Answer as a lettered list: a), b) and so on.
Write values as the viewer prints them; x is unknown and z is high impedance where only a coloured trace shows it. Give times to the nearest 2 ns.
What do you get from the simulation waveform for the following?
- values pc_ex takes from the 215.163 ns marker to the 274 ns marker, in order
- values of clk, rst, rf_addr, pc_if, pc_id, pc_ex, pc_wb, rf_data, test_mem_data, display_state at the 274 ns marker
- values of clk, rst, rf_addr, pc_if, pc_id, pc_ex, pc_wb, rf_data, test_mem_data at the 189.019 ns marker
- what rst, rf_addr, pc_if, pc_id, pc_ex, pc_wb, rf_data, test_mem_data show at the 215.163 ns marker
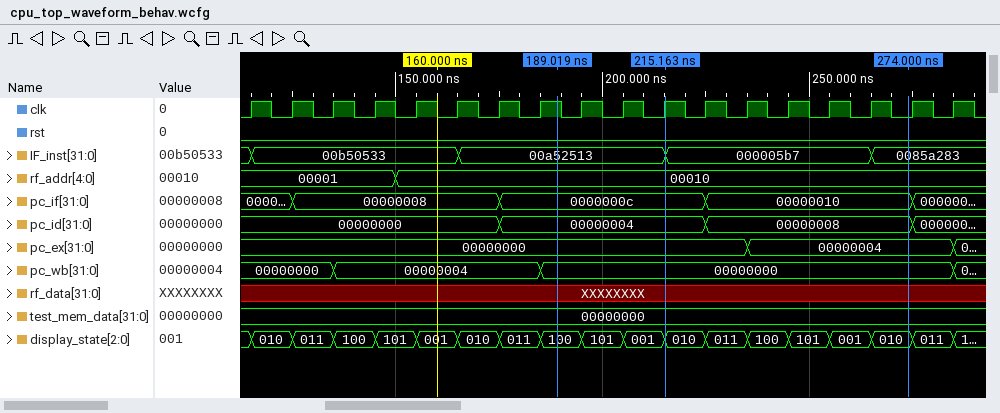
a) 00000000, 00000004
b) clk=0, rst=0, rf_addr=00010, pc_if=00000010, pc_id=00000008, pc_ex=00000004, pc_wb=00000000, rf_data=XXXXXXXX, test_mem_data=00000000, display_state=010
c) clk=1, rst=0, rf_addr=00010, pc_if=0000000c, pc_id=00000004, pc_ex=00000000, pc_wb=00000000, rf_data=XXXXXXXX, test_mem_data=00000000
d) rst=0, rf_addr=00010, pc_if=0000000c, pc_id=00000004, pc_ex=00000000, pc_wb=00000000, rf_data=XXXXXXXX, test_mem_data=00000000
